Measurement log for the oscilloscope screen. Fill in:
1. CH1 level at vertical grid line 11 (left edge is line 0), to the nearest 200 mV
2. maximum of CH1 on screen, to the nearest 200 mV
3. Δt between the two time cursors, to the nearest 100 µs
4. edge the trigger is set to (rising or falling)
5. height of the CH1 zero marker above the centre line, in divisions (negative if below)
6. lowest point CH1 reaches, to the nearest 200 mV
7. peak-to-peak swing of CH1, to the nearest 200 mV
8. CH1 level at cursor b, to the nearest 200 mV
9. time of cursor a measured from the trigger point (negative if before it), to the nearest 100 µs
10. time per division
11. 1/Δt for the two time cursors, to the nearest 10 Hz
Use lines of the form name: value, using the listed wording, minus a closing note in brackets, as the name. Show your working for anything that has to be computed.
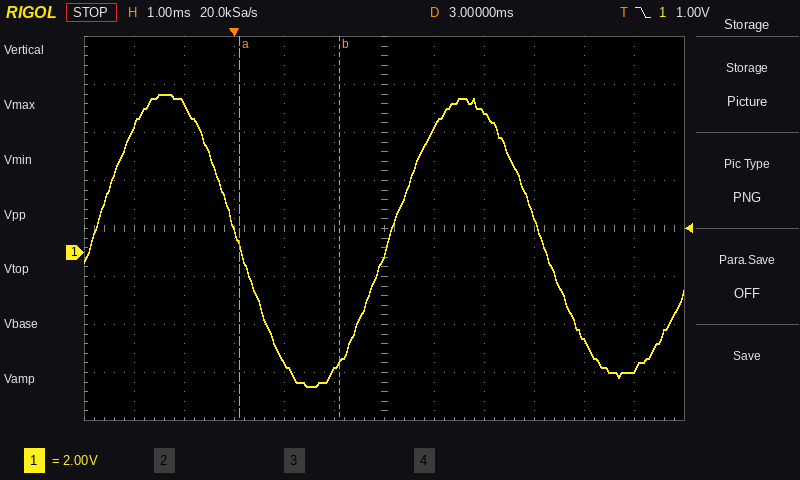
CH1 level at vertical grid line 11 (left edge is line 0), to the nearest 200 mV: -4.8 V
maximum of CH1 on screen, to the nearest 200 mV: 6.6 V
Δt between the two time cursors, to the nearest 100 µs: 2.0 ms
edge the trigger is set to: falling
height of the CH1 zero marker above the centre line, in divisions: -0.5 div
lowest point CH1 reaches, to the nearest 200 mV: -5.6 V
peak-to-peak swing of CH1, to the nearest 200 mV: 6.6 V − (-5.6 V) = 12.2 V
CH1 level at cursor b, to the nearest 200 mV: -4.6 V
time of cursor a measured from the trigger point (negative if before it), to the nearest 100 µs: +100 µs
time per division: 1 ms
1/Δt for the two time cursors, to the nearest 10 Hz: 1 / 2.0 ms ≈ 500 Hz
